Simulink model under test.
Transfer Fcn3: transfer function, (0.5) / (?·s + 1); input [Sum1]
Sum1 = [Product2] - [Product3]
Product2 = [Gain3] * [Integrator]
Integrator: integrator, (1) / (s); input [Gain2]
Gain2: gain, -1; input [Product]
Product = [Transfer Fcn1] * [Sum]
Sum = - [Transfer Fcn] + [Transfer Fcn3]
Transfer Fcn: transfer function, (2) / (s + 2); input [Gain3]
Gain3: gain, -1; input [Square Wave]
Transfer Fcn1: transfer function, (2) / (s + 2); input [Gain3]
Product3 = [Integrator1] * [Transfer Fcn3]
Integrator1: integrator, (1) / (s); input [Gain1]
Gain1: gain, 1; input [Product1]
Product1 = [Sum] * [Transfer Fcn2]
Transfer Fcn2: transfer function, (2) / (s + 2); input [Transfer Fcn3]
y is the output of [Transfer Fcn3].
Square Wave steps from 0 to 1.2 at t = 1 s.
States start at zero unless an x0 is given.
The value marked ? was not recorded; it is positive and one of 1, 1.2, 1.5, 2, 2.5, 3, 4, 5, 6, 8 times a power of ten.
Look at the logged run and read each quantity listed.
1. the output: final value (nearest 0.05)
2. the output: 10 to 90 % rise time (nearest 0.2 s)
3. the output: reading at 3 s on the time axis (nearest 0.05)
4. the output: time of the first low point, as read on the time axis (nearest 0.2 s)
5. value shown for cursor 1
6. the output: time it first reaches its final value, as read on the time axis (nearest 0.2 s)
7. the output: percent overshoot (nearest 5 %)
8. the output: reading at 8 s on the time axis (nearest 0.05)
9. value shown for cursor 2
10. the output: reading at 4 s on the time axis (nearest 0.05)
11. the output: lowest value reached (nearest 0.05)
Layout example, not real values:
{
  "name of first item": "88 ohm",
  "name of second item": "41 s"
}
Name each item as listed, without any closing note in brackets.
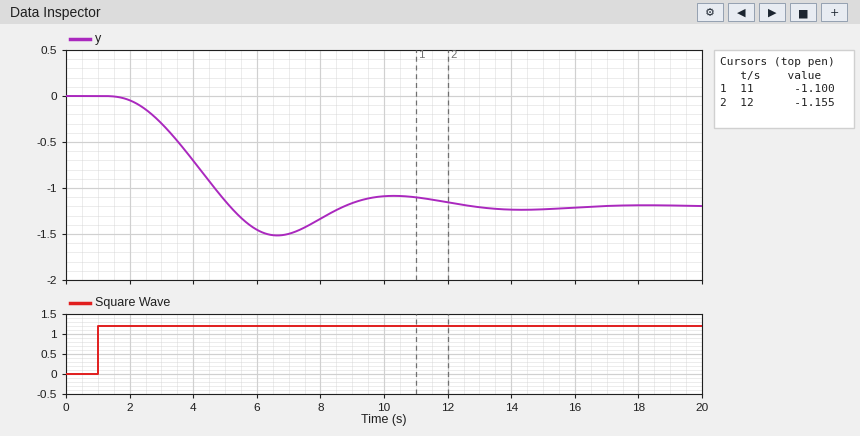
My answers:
{
  "the output: final value": "-1.20",
  "the output: 10 to 90 % rise time": "2.4 s",
  "the output: reading at 3 s on the time axis": "-0.30",
  "the output: time of the first low point, as read on the time axis": "6.6 s",
  "value shown for cursor 1": "-1.100",
  "the output: time it first reaches its final value, as read on the time axis": "5.2 s",
  "the output: percent overshoot": "25 %",
  "the output: reading at 8 s on the time axis": "-1.35",
  "value shown for cursor 2": "-1.155",
  "the output: reading at 4 s on the time axis": "-0.70",
  "the output: lowest value reached": "-1.50"
}
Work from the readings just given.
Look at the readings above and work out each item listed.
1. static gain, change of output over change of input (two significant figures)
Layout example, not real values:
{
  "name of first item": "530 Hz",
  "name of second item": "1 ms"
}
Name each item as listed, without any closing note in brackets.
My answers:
{
  "static gain, change of output over change of input": "-1.0"
}
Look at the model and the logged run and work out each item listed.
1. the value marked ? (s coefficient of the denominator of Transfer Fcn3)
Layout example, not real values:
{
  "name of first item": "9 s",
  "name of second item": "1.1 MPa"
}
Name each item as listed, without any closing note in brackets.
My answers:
{
  "the value marked ?": "2"
}
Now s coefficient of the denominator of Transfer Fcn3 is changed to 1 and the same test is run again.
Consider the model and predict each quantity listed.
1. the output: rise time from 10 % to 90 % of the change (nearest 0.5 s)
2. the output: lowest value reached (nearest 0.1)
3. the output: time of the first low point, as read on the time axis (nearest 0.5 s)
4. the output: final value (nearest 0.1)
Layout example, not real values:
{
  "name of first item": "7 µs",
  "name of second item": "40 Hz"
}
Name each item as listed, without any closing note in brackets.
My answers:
{
  "the output: rise time from 10 % to 90 % of the change": "2.0 s",
  "the output: lowest value reached": "-1.4",
  "the output: time of the first low point, as read on the time axis": "5.5 s",
  "the output: final value": "-1.2"
}
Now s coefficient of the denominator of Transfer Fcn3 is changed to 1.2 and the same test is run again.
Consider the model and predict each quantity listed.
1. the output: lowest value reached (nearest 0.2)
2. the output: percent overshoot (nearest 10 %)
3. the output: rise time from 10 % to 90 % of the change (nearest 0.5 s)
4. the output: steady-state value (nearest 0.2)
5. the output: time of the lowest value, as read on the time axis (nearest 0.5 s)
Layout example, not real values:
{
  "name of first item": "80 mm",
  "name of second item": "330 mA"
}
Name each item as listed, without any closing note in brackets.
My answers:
{
  "the output: lowest value reached": "-1.4",
  "the output: percent overshoot": "20 %",
  "the output: rise time from 10 % to 90 % of the change": "2.0 s",
  "the output: steady-state value": "-1.2",
  "the output: time of the lowest value, as read on the time axis": "6.0 s"
}
